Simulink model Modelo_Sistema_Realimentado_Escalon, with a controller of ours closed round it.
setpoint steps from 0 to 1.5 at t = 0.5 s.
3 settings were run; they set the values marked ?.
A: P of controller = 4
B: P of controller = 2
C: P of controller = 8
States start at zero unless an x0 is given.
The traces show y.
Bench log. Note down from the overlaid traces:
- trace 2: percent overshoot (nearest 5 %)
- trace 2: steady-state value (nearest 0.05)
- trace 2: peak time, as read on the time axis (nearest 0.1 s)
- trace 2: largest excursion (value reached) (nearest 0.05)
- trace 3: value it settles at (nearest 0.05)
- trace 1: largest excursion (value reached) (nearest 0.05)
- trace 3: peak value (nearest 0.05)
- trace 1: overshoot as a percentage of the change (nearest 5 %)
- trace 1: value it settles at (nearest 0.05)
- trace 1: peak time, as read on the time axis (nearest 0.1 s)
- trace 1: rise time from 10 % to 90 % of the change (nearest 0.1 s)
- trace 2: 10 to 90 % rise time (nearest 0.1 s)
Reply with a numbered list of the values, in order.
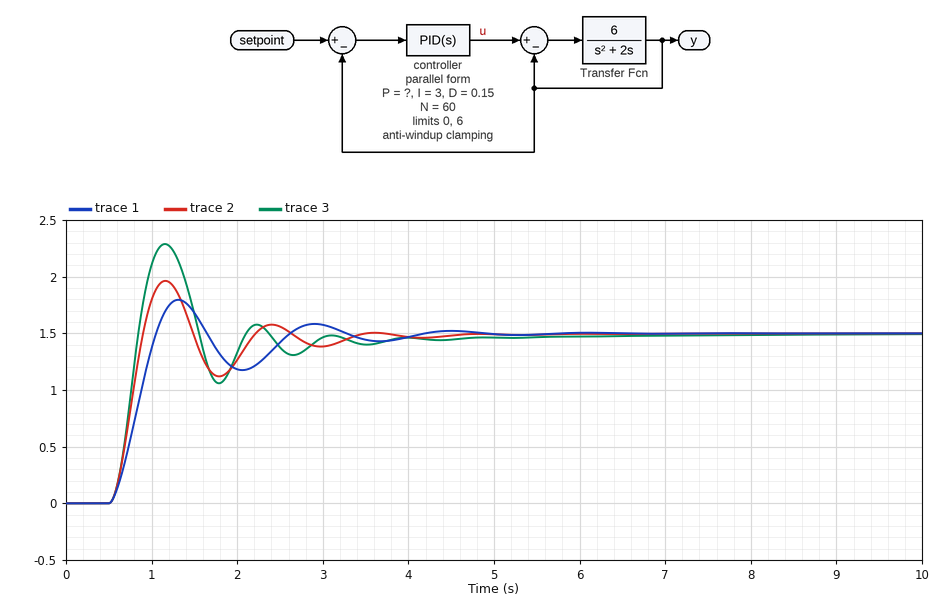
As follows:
1. 30 %
2. 1.50
3. 1.2 s
4. 1.95
5. 1.50
6. 1.80
7. 2.30
8. 20 %
9. 1.50
10. 1.3 s
11. 0.4 s
12. 0.3 s
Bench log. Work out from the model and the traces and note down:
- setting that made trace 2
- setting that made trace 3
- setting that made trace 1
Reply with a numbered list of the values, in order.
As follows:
1. A
2. C
3. B
